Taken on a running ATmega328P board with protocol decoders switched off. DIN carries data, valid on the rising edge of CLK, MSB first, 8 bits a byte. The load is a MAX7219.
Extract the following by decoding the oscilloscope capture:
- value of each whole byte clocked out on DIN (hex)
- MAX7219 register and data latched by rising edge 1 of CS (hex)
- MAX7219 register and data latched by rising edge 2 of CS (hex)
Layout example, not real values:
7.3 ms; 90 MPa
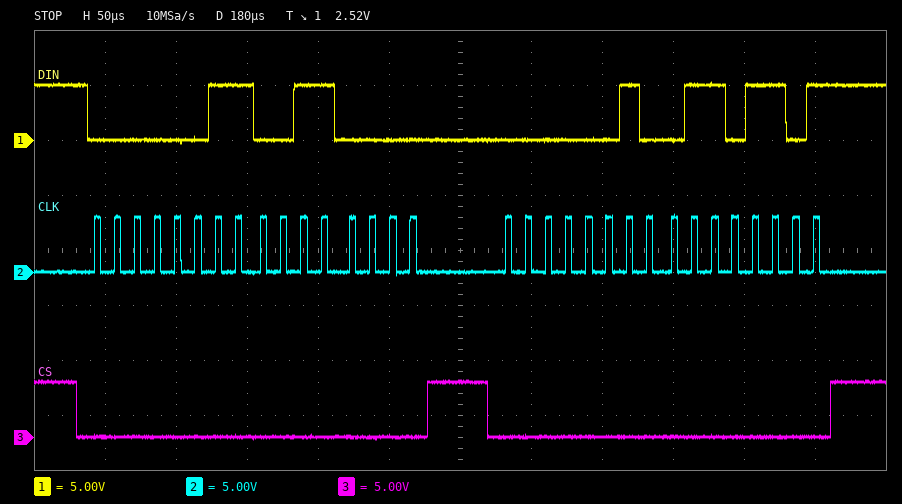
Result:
03 30 02 6D; register 0x3, data 0x30; register 0x2, data 0x6D
